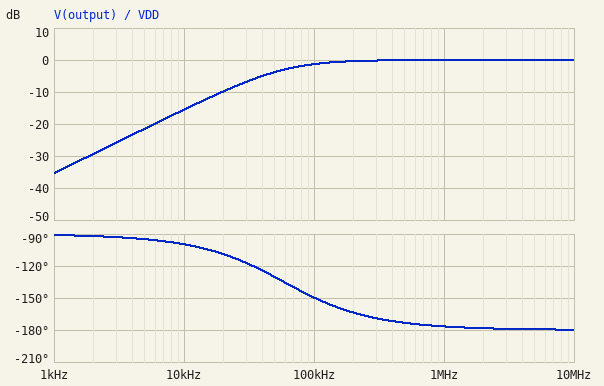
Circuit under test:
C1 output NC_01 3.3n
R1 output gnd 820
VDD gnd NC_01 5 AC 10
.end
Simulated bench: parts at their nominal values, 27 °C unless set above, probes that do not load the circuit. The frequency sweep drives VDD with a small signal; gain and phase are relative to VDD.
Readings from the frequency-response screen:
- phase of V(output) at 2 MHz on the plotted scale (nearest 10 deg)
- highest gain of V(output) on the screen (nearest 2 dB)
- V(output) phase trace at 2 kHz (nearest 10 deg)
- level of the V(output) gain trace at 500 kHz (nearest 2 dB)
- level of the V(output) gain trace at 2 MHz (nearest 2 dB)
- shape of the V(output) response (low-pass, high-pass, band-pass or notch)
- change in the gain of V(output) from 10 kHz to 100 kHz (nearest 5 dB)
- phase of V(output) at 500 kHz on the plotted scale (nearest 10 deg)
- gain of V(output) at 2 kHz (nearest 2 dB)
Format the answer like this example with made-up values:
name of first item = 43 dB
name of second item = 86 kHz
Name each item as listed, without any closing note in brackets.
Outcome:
phase of V(output) at 2 MHz on the plotted scale = -180 deg
highest gain of V(output) on the screen = 0 dB
V(output) phase trace at 2 kHz = -90 deg
level of the V(output) gain trace at 500 kHz = 0 dB
level of the V(output) gain trace at 2 MHz = 0 dB
shape of the V(output) response = high-pass
change in the gain of V(output) from 10 kHz to 100 kHz = 15 dB
phase of V(output) at 500 kHz on the plotted scale = -170 deg
gain of V(output) at 2 kHz = -30 dB
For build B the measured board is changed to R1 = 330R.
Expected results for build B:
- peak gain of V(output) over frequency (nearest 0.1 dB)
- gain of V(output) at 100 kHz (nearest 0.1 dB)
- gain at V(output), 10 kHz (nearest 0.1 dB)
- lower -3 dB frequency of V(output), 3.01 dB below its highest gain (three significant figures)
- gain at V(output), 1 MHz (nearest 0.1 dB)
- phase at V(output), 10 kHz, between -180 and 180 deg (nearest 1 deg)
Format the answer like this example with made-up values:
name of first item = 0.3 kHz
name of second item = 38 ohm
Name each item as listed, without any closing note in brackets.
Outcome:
peak gain of V(output) over frequency = 0 dB
gain of V(output) at 100 kHz = -5.0 dB
gain at V(output), 10 kHz = -23.3 dB
lower -3 dB frequency of V(output), 3.01 dB below its highest gain = 146 kHz
gain at V(output), 1 MHz = -0.1 dB
phase at V(output), 10 kHz, between -180 and 180 deg = -94 deg
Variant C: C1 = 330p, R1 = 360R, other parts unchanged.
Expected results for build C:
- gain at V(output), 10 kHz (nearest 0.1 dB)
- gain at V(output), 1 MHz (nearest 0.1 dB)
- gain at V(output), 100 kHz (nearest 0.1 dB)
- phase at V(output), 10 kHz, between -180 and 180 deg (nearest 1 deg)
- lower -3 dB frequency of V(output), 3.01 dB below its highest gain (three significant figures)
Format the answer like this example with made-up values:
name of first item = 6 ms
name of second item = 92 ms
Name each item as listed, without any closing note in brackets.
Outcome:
gain at V(output), 10 kHz = -42.5 dB
gain at V(output), 1 MHz = -4.5 dB
gain at V(output), 100 kHz = -22.6 dB
phase at V(output), 10 kHz, between -180 and 180 deg = -90 deg
lower -3 dB frequency of V(output), 3.01 dB below its highest gain = 1.34 MHz
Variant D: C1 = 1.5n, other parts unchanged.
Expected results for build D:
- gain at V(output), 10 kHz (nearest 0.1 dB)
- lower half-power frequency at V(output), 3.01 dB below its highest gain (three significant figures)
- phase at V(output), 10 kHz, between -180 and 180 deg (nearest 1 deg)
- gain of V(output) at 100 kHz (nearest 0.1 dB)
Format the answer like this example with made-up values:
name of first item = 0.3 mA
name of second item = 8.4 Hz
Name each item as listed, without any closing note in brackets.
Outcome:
gain at V(output), 10 kHz = -22.3 dB
lower half-power frequency at V(output), 3.01 dB below its highest gain = 129 kHz
phase at V(output), 10 kHz, between -180 and 180 deg = -94 deg
gain of V(output) at 100 kHz = -4.3 dB
